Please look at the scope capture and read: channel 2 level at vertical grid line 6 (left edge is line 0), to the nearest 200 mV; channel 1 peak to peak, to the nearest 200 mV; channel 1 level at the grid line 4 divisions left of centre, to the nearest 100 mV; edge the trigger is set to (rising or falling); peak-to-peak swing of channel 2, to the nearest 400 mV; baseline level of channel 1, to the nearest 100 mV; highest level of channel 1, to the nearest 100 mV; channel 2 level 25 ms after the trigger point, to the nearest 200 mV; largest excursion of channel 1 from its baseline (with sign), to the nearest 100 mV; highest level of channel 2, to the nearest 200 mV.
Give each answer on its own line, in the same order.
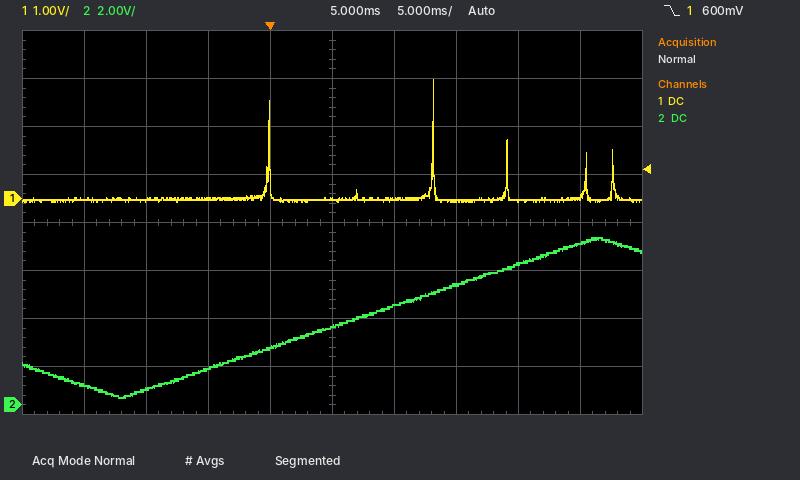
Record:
4.2 V
2.6 V
0.0 V
falling
6.8 V
0.0 V
2.5 V
6.8 V
+2.5 V
7.0 V
